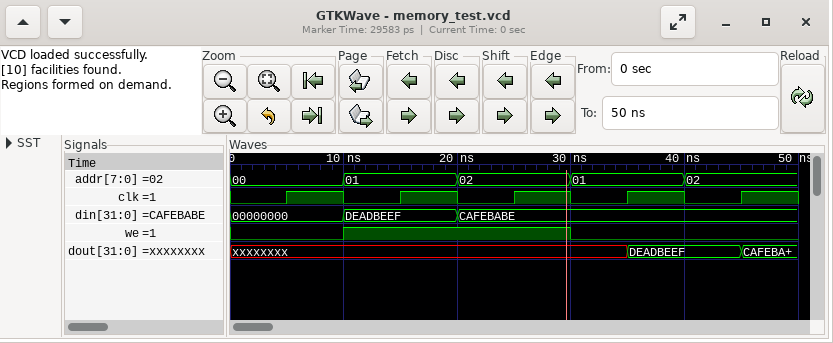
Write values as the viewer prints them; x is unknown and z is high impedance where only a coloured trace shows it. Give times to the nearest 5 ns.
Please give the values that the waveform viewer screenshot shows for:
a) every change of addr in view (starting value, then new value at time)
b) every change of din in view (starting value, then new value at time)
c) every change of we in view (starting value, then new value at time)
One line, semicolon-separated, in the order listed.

00, 01 at 10 ns, 02 at 20 ns, 01 at 30 ns, 02 at 40 ns; 00000000, DEADBEEF at 10 ns, CAFEBABE at 20 ns; 0, 1 at 10 ns, 0 at 30 ns
